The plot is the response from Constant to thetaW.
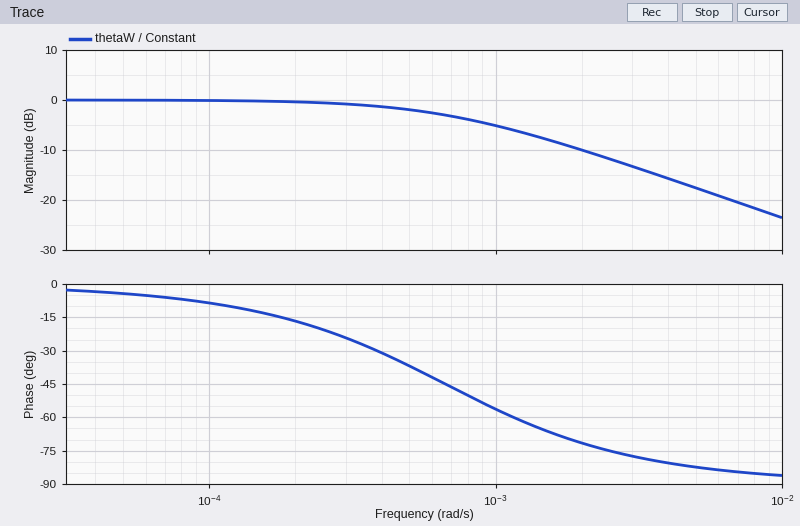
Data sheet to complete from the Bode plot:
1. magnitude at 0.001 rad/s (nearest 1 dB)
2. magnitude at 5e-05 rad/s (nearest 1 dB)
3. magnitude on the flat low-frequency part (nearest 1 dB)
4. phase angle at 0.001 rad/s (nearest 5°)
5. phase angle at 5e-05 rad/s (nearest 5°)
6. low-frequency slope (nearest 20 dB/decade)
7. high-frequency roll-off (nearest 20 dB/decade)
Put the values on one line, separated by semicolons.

-5 dB; 0 dB; 0 dB; -55°; -5°; 0 dB/decade; -20 dB/decade
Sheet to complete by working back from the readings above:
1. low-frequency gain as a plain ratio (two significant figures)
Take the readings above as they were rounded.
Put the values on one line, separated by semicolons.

1.0
